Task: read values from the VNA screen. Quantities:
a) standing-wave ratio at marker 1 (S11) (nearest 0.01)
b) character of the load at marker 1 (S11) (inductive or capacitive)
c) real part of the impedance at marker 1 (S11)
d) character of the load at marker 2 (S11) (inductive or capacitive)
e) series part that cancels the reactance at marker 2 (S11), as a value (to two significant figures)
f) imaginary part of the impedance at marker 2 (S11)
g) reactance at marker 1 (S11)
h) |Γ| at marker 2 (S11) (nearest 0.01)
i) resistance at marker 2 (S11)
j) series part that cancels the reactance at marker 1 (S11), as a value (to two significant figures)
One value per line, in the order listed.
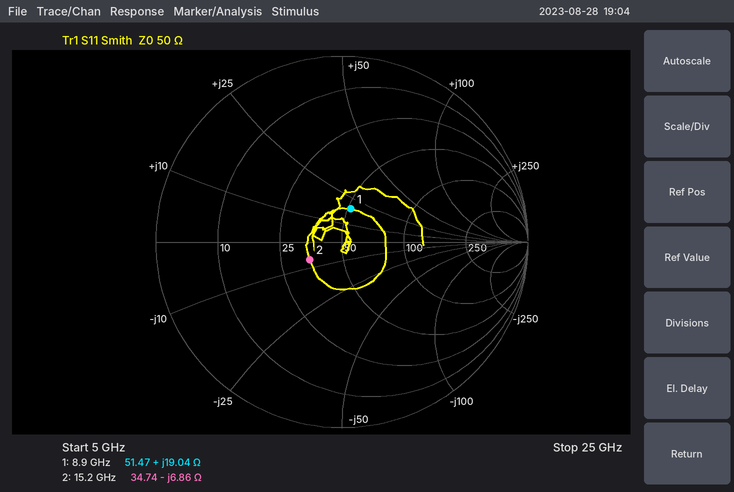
1.45
inductive
51.47 Ω
capacitive
72 pH
-6.86 Ω
+19.04 Ω
0.20
34.74 Ω
940 fF
